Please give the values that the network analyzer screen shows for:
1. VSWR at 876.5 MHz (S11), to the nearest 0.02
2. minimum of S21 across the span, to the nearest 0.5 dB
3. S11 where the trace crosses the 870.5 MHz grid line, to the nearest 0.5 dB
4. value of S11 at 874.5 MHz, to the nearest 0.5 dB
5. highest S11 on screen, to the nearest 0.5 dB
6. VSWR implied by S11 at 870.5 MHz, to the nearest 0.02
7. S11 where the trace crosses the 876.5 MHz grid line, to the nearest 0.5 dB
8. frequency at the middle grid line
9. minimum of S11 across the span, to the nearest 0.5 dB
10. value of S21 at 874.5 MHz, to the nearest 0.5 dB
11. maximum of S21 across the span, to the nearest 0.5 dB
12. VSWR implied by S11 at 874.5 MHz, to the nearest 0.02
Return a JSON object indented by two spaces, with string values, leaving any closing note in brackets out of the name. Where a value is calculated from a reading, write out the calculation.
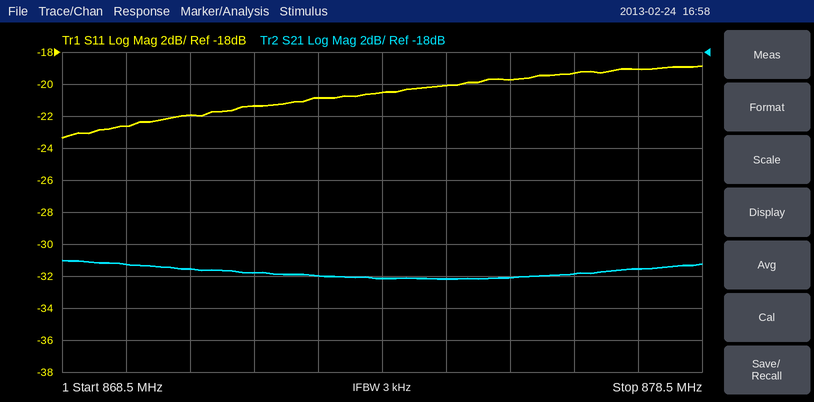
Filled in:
{
  "VSWR at 876.5 MHz (S11), to the nearest 0.02": "|Γ| = 10^(-19.5/20) = 0.1059; VSWR = (1 + 0.1059)/(1 − 0.1059) ≈ 1.24",
  "minimum of S21 across the span, to the nearest 0.5 dB": "-32.0 dB",
  "S11 where the trace crosses the 870.5 MHz grid line, to the nearest 0.5 dB": "-22.0 dB",
  "value of S11 at 874.5 MHz, to the nearest 0.5 dB": "-20.0 dB",
  "highest S11 on screen, to the nearest 0.5 dB": "-19.0 dB",
  "VSWR implied by S11 at 870.5 MHz, to the nearest 0.02": "|Γ| = 10^(-22/20) = 0.0794; VSWR = (1 + 0.0794)/(1 − 0.0794) ≈ 1.17, so 1.18 to the nearest 0.02",
  "S11 where the trace crosses the 876.5 MHz grid line, to the nearest 0.5 dB": "-19.5 dB",
  "frequency at the middle grid line": "873.5 MHz",
  "minimum of S11 across the span, to the nearest 0.5 dB": "-23.5 dB",
  "value of S21 at 874.5 MHz, to the nearest 0.5 dB": "-32.0 dB",
  "maximum of S21 across the span, to the nearest 0.5 dB": "-31.0 dB",
  "VSWR implied by S11 at 874.5 MHz, to the nearest 0.02": "|Γ| = 10^(-20/20) = 0.1000; VSWR = (1 + 0.1000)/(1 − 0.1000) ≈ 1.22"
}
